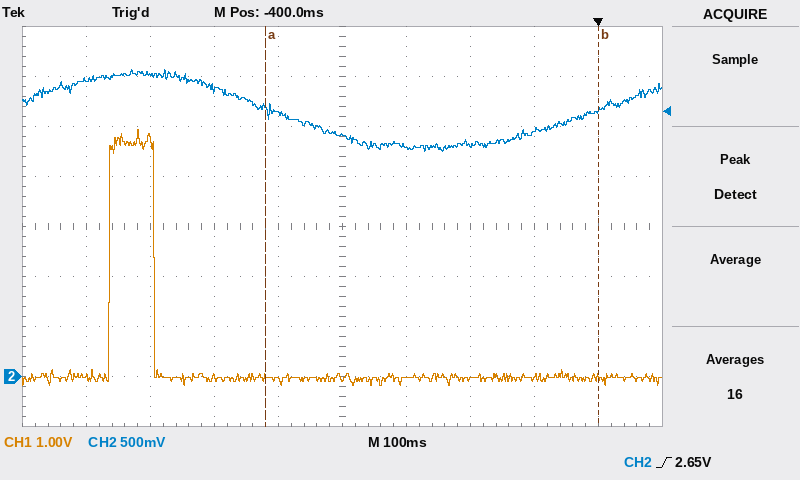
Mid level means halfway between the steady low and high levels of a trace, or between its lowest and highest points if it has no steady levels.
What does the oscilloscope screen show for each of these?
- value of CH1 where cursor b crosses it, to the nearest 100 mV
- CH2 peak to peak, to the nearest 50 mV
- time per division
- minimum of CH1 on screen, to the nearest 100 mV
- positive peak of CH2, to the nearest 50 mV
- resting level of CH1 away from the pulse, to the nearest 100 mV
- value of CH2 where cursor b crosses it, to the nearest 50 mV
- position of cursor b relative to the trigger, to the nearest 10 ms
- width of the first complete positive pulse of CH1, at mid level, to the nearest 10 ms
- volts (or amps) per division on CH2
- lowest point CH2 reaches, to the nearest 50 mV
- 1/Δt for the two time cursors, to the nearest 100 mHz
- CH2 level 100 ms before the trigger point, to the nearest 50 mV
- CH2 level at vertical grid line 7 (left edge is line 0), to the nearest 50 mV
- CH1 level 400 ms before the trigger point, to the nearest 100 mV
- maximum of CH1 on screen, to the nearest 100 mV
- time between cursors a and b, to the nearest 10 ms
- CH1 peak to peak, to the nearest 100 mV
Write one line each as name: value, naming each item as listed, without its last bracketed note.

value of CH1 where cursor b crosses it, to the nearest 100 mV: 0.0 V
CH2 peak to peak, to the nearest 50 mV: 800 mV
time per division: 100 ms
minimum of CH1 on screen, to the nearest 100 mV: -200 mV
positive peak of CH2, to the nearest 50 mV: 3.05 V
resting level of CH1 away from the pulse, to the nearest 100 mV: 0.0 V
value of CH2 where cursor b crosses it, to the nearest 50 mV: 2.65 V
position of cursor b relative to the trigger, to the nearest 10 ms: 0 ms
width of the first complete positive pulse of CH1, at mid level, to the nearest 10 ms: 70 ms
volts (or amps) per division on CH2: 500 mV
lowest point CH2 reaches, to the nearest 50 mV: 2.25 V
1/Δt for the two time cursors, to the nearest 100 mHz: 1.9 Hz
CH2 level 100 ms before the trigger point, to the nearest 50 mV: 2.45 V
CH2 level at vertical grid line 7 (left edge is line 0), to the nearest 50 mV: 2.30 V
CH1 level 400 ms before the trigger point, to the nearest 100 mV: 0.0 V
maximum of CH1 on screen, to the nearest 100 mV: 4.9 V
time between cursors a and b, to the nearest 10 ms: 520 ms
CH1 peak to peak, to the nearest 100 mV: 5.1 V
